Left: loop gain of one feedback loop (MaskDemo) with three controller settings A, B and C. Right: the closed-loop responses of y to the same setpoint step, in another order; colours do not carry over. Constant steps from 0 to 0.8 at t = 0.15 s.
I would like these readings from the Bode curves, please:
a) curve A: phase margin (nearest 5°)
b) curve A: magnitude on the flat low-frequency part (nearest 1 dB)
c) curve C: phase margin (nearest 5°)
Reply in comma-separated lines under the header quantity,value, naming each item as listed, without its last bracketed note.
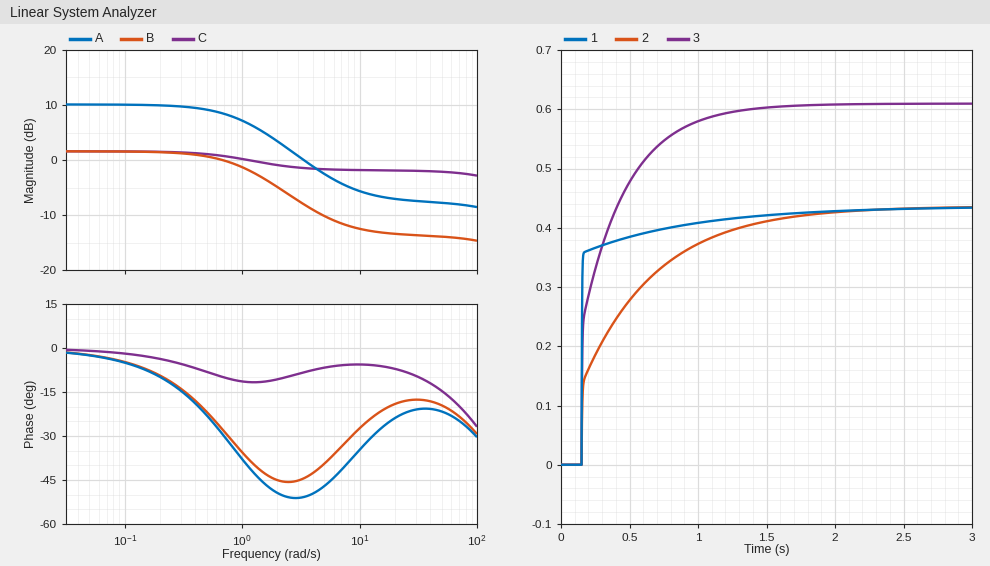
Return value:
quantity,value
curve A: phase margin,130°
curve A: magnitude on the flat low-frequency part,10 dB
curve C: phase margin,170°
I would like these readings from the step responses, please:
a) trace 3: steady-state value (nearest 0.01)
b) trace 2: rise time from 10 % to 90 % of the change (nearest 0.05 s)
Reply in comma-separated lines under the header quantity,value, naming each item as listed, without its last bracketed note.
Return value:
quantity,value
trace 3: steady-state value,0.61
trace 2: rise time from 10 % to 90 % of the change,1.05 s
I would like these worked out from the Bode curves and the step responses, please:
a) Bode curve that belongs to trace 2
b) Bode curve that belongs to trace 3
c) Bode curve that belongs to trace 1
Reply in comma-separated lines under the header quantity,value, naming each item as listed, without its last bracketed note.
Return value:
quantity,value
Bode curve that belongs to trace 2,B
Bode curve that belongs to trace 3,A
Bode curve that belongs to trace 1,C
